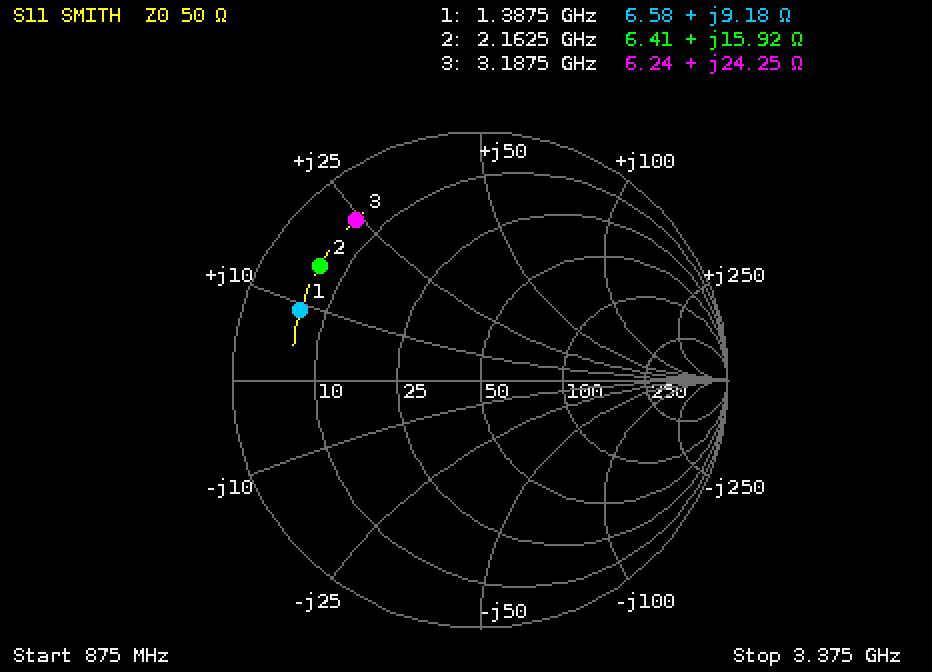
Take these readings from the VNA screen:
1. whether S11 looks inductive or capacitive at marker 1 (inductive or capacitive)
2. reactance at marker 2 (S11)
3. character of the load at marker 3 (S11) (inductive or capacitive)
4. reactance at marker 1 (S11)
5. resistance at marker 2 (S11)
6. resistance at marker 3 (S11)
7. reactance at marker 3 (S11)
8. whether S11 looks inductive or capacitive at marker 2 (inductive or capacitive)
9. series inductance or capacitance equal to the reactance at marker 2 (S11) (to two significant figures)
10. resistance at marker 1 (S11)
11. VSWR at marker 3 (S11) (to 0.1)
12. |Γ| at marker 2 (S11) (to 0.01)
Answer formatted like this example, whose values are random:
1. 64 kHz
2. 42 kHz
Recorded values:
1. inductive
2. +15.92 Ω
3. inductive
4. +9.18 Ω
5. 6.41 Ω
6. 6.24 Ω
7. +24.25 Ω
8. inductive
9. 1.2 nH
10. 6.58 Ω
11. 9.9
12. 0.79
